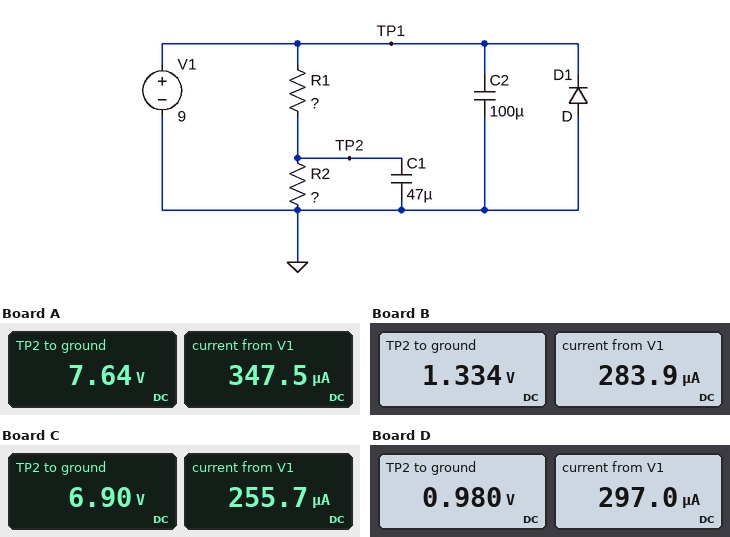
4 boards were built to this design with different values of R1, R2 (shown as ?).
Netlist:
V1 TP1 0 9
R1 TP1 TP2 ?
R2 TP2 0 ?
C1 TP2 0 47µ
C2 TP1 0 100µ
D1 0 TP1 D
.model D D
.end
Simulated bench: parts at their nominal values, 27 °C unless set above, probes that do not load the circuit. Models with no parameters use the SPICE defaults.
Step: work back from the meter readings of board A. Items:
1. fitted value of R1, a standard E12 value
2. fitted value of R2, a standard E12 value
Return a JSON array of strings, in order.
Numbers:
["3.9 kΩ", "22 kΩ"]
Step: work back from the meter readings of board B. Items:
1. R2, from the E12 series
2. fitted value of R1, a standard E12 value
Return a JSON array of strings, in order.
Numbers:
["4.7 kΩ", "27 kΩ"]
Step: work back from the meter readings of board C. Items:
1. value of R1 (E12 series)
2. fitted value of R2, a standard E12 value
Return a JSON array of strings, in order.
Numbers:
["8.2 kΩ", "27 kΩ"]
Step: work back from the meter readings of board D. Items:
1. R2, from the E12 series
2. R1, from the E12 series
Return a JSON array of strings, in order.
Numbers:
["3.3 kΩ", "27 kΩ"]
